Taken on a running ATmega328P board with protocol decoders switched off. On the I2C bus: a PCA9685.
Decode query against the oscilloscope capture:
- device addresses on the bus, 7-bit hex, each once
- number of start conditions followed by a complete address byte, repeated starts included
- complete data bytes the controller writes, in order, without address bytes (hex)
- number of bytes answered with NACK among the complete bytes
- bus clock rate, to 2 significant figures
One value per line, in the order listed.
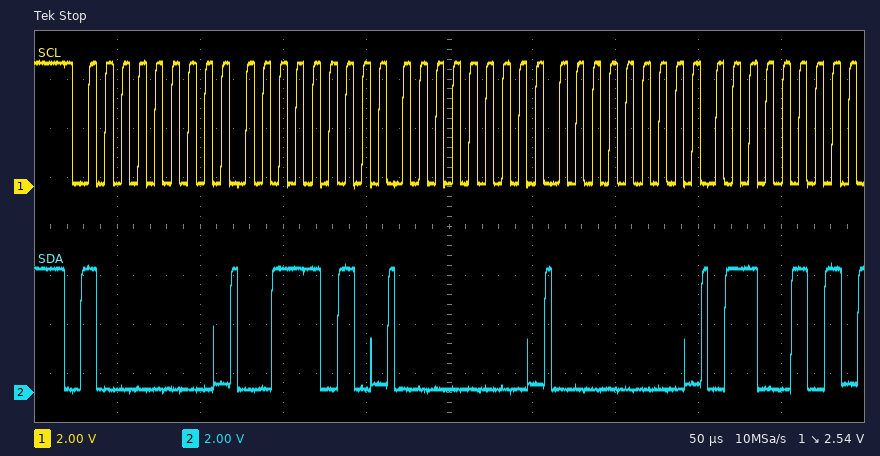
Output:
0x40
1
3A 00 00 65
0
100 kHz
